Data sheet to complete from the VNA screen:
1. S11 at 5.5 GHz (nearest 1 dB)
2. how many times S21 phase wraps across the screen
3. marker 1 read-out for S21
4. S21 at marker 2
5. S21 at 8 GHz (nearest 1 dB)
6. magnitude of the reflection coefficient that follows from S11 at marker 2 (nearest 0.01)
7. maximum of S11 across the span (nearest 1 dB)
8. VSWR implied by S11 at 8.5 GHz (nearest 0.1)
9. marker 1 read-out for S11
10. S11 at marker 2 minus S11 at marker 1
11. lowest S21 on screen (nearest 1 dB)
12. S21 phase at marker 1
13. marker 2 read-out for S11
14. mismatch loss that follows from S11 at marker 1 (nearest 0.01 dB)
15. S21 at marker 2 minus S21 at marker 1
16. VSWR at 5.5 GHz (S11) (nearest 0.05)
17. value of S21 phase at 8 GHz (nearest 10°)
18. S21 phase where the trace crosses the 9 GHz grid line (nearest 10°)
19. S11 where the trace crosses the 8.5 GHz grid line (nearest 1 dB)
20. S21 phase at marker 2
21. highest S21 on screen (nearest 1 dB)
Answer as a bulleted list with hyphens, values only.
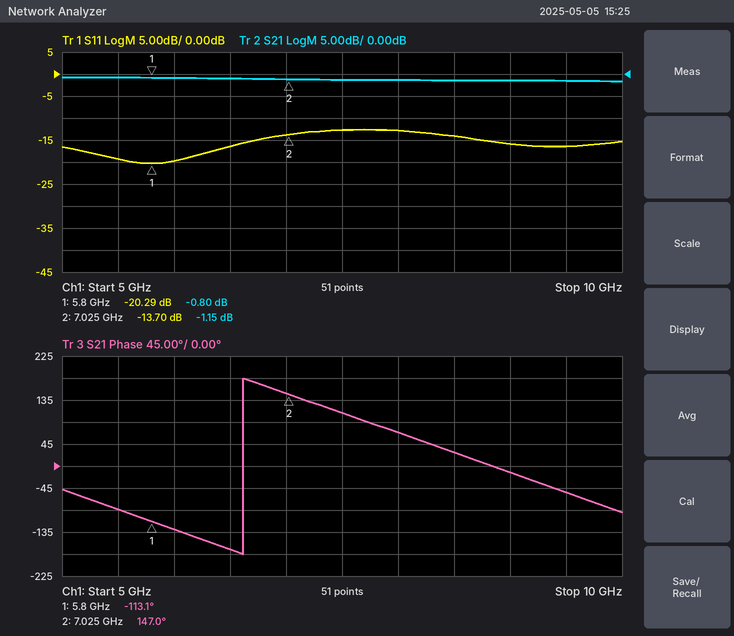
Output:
- -19 dB
- 1
- -0.80 dB
- -1.15 dB
- -1 dB
- 0.21
- -13 dB
- 1.5
- -20.29 dB
- 6.59 dB
- -2 dB
- -113.1°
- -13.70 dB
- 0.04 dB
- -0.35 dB
- 1.25
- 70°
- -10°
- -14 dB
- 147.0°
- -1 dB
